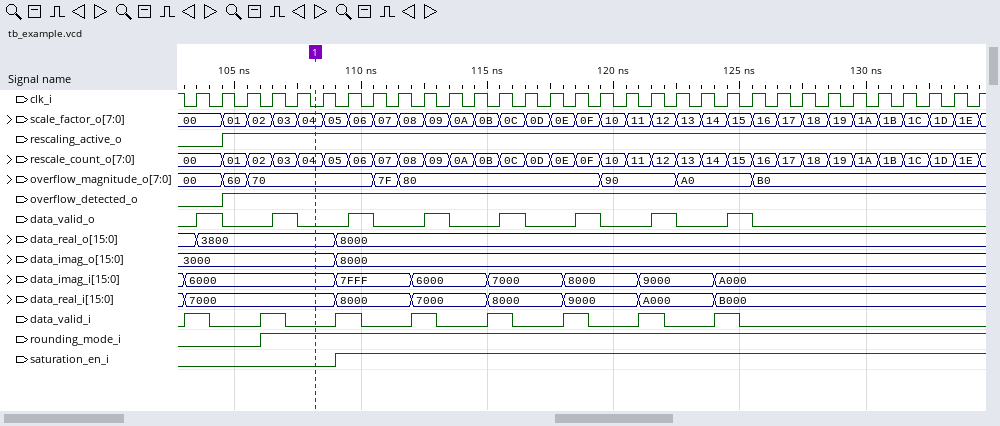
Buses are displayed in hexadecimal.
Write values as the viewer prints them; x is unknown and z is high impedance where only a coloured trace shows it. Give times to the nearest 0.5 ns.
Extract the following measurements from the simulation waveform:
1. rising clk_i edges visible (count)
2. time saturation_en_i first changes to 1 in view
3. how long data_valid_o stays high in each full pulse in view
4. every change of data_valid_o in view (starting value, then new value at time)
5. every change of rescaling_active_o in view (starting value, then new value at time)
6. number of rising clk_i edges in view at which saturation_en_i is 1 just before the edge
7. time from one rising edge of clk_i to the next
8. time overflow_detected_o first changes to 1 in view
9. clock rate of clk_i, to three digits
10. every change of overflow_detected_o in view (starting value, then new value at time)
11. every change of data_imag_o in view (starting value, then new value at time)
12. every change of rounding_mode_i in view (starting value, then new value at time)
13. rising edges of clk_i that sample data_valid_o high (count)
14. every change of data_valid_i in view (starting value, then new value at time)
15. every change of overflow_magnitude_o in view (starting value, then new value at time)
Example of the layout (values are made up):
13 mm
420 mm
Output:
32
109 ns
1 ns, 1 ns, 1 ns, 1 ns, 1 ns, 1 ns, 1 ns, 1 ns
0, 1 at 103.5 ns, 0 at 104.5 ns, 1 at 106.5 ns, 0 at 107.5 ns, 1 at 109.5 ns, 0 at 110.5 ns, 1 at 112.5 ns, 0 at 113.5 ns, 1 at 115.5 ns, 0 at 116.5 ns, 1 at 118.5 ns, 0 at 119.5 ns, 1 at 121.5 ns, 0 at 122.5 ns, 1 at 124.5 ns, 0 at 125.5 ns
0, 1 at 104.5 ns
26
1 ns
104.5 ns
1.00 GHz
0, 1 at 104.5 ns
3000, 8000 at 109 ns
0, 1 at 106 ns
8
0, 1 at 103 ns, 0 at 104 ns, 1 at 106 ns, 0 at 107 ns, 1 at 109 ns, 0 at 110 ns, 1 at 112 ns, 0 at 113 ns, 1 at 115 ns, 0 at 116 ns, 1 at 118 ns, 0 at 119 ns, 1 at 121 ns, 0 at 122 ns, 1 at 124 ns, 0 at 125 ns
00, 60 at 104.5 ns, 70 at 105.5 ns, 7F at 110.5 ns, 80 at 111.5 ns, 90 at 119.5 ns, A0 at 122.5 ns, B0 at 125.5 ns
